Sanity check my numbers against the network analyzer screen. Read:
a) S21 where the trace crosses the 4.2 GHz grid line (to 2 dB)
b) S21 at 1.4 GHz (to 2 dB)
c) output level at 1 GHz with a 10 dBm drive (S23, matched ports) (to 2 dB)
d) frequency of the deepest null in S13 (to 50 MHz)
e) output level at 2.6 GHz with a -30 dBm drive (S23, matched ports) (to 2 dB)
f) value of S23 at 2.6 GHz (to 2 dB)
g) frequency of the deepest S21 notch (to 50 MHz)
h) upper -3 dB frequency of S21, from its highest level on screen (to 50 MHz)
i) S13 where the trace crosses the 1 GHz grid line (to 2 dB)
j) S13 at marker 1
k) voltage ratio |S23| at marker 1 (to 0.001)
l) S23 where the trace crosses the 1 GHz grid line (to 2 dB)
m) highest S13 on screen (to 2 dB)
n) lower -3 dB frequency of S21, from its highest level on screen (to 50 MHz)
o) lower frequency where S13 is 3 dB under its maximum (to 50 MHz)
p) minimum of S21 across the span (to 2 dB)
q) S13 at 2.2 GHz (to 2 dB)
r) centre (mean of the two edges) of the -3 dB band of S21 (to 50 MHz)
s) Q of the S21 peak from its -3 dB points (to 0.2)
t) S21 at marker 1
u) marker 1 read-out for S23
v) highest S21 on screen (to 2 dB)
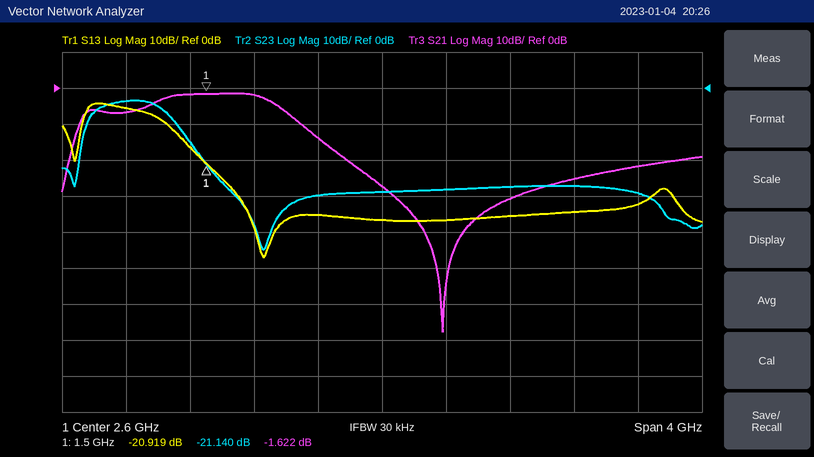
-22 dB
-2 dB
6 dBm
1.85 GHz
-58 dBm
-28 dB
3.00 GHz
1.95 GHz
-6 dB
-20.919 dB
0.088
-4 dB
-4 dB
1.15 GHz
750 MHz
-68 dB
-36 dB
1.55 GHz
2.0
-1.622 dB
-21.140 dB
-2 dB
